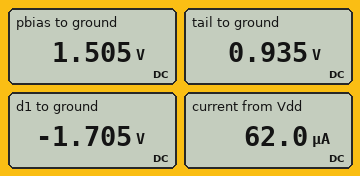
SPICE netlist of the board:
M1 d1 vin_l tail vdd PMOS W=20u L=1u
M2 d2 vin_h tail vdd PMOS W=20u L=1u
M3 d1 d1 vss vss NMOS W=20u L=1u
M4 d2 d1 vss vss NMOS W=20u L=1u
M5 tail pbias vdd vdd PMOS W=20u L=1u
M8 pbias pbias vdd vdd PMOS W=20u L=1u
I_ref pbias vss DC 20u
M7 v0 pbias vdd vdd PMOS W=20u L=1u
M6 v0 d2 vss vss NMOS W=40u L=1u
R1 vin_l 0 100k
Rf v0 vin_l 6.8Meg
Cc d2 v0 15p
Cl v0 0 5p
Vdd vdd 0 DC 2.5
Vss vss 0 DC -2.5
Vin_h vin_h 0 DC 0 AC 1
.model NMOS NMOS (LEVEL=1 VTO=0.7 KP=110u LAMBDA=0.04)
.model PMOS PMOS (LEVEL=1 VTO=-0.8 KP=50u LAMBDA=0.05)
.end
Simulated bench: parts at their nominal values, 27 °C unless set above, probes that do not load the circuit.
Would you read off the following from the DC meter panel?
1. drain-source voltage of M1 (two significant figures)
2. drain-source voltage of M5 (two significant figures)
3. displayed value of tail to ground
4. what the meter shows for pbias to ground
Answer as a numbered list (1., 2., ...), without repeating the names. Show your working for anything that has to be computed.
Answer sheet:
1. -1.705 V - 935 mV = -2.6 V
2. 935 mV - 2.5 V = -1.6 V
3. 0.935 V
4. 1.505 V
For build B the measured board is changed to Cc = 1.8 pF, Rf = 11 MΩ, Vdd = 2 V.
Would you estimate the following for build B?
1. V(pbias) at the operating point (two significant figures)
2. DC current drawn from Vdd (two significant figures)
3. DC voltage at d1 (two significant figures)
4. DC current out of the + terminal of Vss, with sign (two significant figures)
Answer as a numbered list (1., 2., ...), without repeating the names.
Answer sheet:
1. 1.0 V
2. 61 µA
3. -1.7 V
4. -61 µA
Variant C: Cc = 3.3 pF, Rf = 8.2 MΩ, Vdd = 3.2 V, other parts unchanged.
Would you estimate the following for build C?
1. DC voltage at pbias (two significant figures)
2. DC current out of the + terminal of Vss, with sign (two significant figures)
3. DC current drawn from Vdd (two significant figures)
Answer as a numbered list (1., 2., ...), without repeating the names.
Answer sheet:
1. 2.2 V
2. -63 µA
3. 63 µA
